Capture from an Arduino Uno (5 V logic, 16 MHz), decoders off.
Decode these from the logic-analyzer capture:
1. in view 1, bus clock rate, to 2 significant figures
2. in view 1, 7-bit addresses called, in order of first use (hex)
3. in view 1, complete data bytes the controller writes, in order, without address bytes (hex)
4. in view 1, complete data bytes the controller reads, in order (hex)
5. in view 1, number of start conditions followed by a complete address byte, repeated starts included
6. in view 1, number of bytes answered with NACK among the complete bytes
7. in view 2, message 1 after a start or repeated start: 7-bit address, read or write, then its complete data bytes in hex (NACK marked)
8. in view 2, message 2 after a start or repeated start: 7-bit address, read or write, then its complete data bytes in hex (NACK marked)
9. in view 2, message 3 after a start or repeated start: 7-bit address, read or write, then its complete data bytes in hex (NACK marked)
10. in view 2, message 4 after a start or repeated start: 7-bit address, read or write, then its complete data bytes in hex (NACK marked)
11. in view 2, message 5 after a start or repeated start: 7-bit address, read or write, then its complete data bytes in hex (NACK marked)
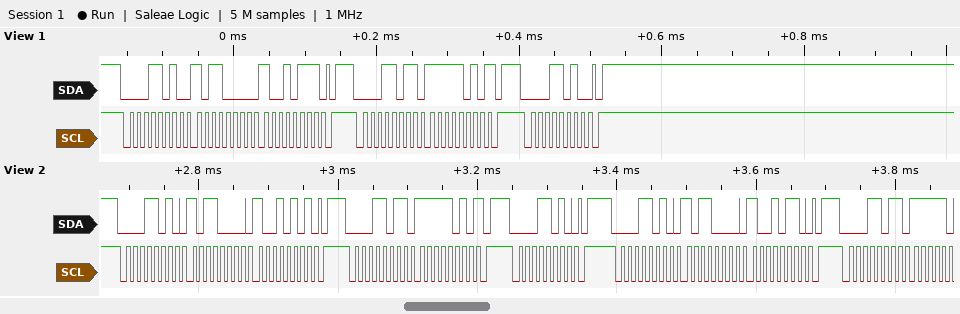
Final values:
100 kHz
0x0D
B0 97
FA
3
1
0x0D write: B0 95
0x0D read: FA NACK
0x0D write
0x0D write: B0 96
0x0D read
